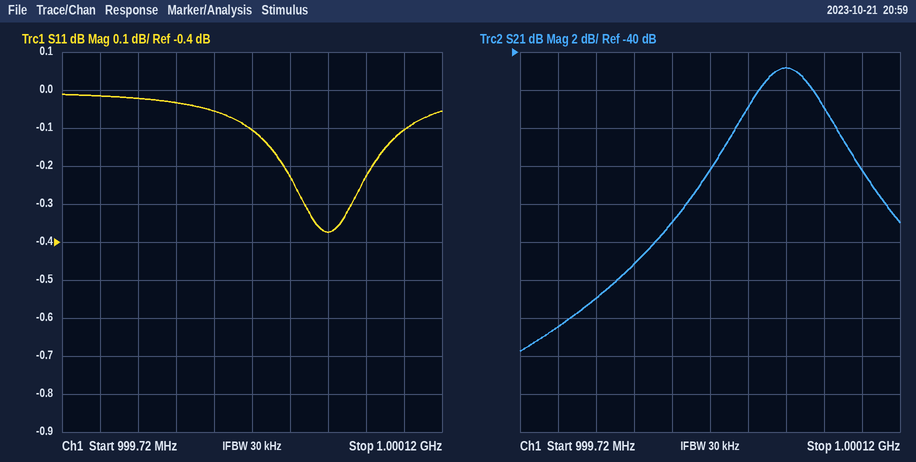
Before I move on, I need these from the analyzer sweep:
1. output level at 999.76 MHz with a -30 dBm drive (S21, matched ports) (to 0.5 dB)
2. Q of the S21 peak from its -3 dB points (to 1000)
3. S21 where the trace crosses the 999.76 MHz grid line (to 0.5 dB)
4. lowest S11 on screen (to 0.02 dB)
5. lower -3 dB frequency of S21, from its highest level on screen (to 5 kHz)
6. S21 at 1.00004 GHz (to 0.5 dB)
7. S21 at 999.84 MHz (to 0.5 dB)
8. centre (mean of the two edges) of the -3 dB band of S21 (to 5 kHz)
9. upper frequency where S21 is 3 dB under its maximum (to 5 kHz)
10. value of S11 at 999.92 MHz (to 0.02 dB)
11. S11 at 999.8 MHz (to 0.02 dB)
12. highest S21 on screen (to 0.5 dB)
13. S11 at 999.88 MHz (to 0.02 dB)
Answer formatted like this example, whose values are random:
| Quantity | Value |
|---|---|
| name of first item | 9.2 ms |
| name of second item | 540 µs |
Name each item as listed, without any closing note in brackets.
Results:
| Quantity | Value |
|---|---|
| output level at 999.76 MHz with a -30 dBm drive (S21, matched ports) | -84.5 dBm |
| Q of the S21 peak from its -3 dB points | 10000 |
| S21 where the trace crosses the 999.76 MHz grid line | -54.5 dB |
| lowest S11 on screen | -0.38 dB |
| lower -3 dB frequency of S21, from its highest level on screen | 999.950 MHz |
| S21 at 1.00004 GHz | -43.0 dB |
| S21 at 999.84 MHz | -51.0 dB |
| centre (mean of the two edges) of the -3 dB band of S21 | 1.000000 GHz |
| upper frequency where S21 is 3 dB under its maximum | 1.000050 GHz |
| value of S11 at 999.92 MHz | -0.10 dB |
| S11 at 999.8 MHz | -0.02 dB |
| highest S21 on screen | -41.0 dB |
| S11 at 999.88 MHz | -0.06 dB |
